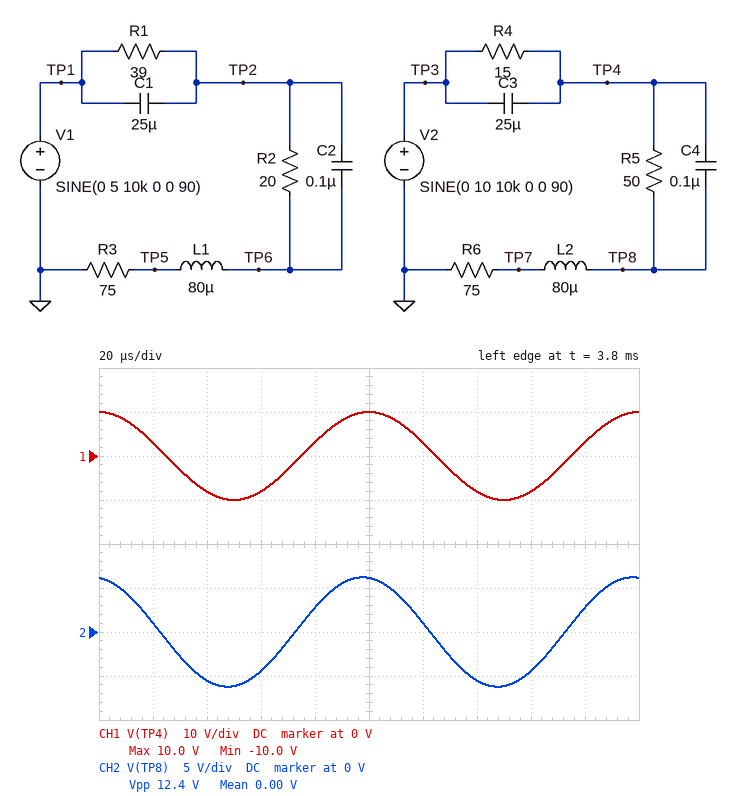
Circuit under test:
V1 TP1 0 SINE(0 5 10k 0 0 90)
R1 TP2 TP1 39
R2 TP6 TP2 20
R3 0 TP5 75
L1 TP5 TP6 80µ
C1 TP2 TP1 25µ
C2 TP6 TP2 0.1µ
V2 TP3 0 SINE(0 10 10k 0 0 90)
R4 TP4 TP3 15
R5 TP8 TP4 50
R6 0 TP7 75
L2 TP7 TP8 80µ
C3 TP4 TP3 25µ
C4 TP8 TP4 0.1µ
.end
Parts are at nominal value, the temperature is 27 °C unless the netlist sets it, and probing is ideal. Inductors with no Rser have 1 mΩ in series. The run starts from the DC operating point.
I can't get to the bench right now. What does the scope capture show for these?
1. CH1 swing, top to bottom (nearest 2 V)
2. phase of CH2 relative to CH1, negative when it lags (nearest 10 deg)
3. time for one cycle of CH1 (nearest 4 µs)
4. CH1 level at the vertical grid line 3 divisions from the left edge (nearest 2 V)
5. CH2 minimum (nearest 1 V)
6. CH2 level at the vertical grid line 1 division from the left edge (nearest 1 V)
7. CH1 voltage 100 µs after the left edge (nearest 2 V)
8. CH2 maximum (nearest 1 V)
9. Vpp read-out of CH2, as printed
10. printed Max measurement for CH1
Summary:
20 V
10 deg
100 µs
-8 V
-6 V
1 V
10 V
6 V
12.4 V
10.0 V
